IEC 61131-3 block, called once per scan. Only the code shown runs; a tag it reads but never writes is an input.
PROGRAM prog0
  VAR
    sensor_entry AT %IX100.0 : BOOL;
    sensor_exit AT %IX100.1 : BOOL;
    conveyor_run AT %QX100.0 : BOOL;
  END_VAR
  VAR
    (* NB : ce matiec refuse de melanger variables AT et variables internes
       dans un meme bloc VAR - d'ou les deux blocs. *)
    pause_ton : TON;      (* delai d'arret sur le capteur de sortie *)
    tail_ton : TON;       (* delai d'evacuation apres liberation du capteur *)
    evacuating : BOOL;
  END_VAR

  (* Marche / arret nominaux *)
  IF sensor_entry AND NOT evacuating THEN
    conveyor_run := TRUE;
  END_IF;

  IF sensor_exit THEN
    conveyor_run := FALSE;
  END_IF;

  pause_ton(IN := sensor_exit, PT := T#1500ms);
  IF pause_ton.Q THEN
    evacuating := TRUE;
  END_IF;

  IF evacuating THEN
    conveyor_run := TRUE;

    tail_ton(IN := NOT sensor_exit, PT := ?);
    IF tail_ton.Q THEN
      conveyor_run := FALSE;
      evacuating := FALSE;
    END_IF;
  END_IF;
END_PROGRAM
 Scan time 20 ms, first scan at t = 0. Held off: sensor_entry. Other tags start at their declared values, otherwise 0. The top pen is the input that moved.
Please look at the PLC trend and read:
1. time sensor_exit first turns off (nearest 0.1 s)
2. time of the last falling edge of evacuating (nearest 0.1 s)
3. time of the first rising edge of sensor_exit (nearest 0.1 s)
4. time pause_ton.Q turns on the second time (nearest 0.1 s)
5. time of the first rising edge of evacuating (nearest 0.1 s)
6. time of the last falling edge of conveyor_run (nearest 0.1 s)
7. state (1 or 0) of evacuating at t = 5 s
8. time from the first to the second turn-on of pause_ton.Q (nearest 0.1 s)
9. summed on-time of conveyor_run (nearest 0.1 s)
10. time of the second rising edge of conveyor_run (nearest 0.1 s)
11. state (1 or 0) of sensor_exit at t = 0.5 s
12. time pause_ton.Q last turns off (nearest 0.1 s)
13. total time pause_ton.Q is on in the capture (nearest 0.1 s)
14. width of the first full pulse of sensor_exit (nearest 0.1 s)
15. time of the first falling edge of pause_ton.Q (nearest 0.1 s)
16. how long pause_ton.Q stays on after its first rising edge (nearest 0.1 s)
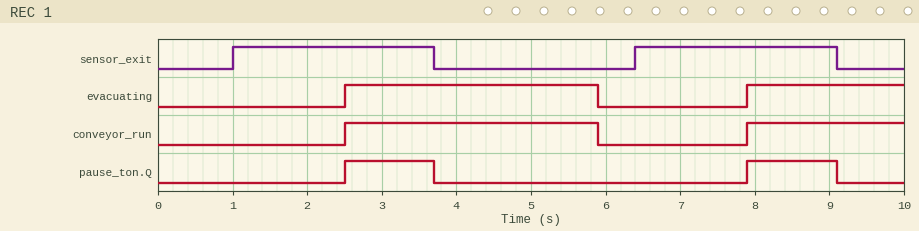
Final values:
3.7 s
5.9 s
1.0 s
7.9 s
2.5 s
5.9 s
1
5.4 s
5.5 s
7.9 s
0
9.1 s
2.4 s
2.7 s
3.7 s
1.2 s
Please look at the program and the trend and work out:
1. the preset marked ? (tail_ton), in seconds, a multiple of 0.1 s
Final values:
2.2 s
